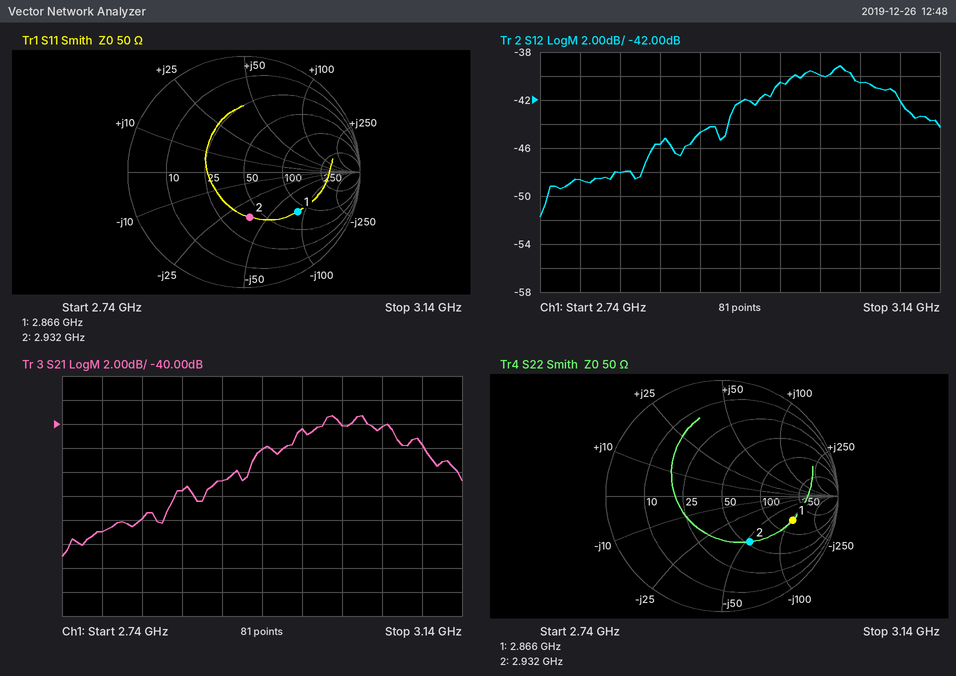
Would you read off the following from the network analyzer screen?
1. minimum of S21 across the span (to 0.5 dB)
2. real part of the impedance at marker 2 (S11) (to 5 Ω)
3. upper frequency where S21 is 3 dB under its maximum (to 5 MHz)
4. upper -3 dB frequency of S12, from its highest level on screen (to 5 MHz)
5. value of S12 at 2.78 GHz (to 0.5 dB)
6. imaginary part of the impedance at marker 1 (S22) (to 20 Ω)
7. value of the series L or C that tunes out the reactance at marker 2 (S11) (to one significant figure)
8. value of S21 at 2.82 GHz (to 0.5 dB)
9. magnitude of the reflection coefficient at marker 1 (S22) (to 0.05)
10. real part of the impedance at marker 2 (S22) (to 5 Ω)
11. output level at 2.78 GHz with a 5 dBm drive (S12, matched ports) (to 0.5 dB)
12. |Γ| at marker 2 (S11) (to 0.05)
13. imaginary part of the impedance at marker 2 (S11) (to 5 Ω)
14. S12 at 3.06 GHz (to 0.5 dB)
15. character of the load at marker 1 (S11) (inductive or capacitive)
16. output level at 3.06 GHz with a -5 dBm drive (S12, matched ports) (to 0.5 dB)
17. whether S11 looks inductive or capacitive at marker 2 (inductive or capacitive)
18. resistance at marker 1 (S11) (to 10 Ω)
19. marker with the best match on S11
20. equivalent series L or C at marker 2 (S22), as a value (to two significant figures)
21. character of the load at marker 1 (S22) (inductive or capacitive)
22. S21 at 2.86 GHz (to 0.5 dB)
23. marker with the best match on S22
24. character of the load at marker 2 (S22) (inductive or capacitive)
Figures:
-51.0 dB
40 Ω
3.105 GHz
3.100 GHz
-48.5 dB
-100 Ω
2 nH
-48.0 dB
0.65
55 Ω
-43.5 dBm
0.40
-35 Ω
-40.5 dB
capacitive
-45.5 dBm
capacitive
80 Ω
marker 2
1.0 pF
capacitive
-45.5 dB
marker 2
capacitive
